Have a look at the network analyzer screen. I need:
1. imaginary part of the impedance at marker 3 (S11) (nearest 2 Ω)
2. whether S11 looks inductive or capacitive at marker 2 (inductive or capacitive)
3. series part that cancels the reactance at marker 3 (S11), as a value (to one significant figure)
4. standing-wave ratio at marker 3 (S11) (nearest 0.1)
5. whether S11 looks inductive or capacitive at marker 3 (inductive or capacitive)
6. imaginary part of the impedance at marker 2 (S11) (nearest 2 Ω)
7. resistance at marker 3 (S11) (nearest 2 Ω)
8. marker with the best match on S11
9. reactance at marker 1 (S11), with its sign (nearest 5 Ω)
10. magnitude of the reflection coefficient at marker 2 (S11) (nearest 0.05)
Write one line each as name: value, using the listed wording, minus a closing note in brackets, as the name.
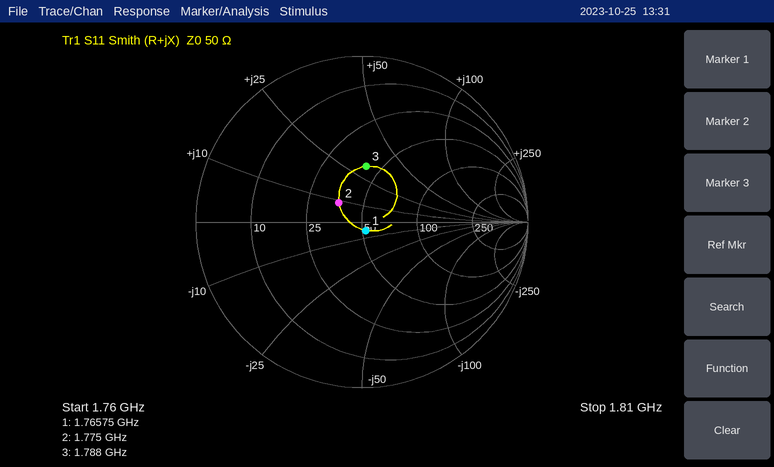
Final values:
imaginary part of the impedance at marker 3 (S11): +32 Ω
whether S11 looks inductive or capacitive at marker 2: inductive
series part that cancels the reactance at marker 3 (S11), as a value: 3 pF
standing-wave ratio at marker 3 (S11): 2.0
whether S11 looks inductive or capacitive at marker 3: inductive
imaginary part of the impedance at marker 2 (S11): +8 Ω
resistance at marker 3 (S11): 42 Ω
marker with the best match on S11: marker 1
reactance at marker 1 (S11), with its sign: -5 Ω
magnitude of the reflection coefficient at marker 2 (S11): 0.20
